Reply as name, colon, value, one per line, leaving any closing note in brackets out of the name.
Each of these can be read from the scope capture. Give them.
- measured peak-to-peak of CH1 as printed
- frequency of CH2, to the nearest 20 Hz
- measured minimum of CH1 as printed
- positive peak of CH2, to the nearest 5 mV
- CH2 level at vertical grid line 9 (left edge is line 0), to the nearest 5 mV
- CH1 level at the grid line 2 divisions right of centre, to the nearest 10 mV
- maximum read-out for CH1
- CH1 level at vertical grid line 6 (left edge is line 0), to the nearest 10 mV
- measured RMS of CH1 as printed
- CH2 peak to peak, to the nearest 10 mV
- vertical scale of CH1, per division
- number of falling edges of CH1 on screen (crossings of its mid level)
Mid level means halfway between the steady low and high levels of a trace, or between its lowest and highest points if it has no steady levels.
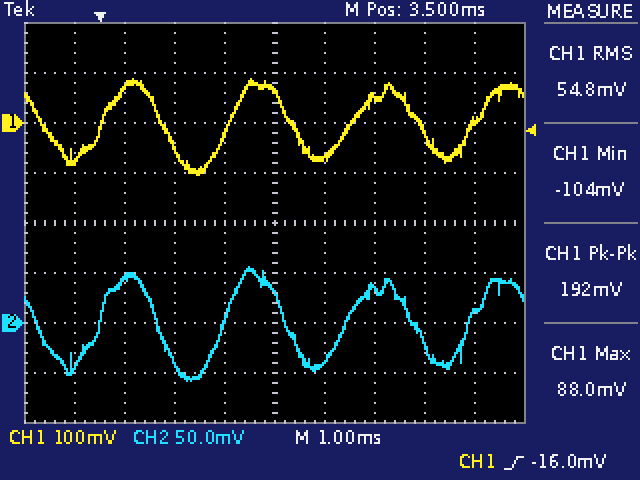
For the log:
measured peak-to-peak of CH1 as printed: 192 mV
frequency of CH2, to the nearest 20 Hz: 400 Hz
measured minimum of CH1 as printed: -104 mV
positive peak of CH2, to the nearest 5 mV: 55 mV
CH2 level at vertical grid line 9 (left edge is line 0), to the nearest 5 mV: 10 mV
CH1 level at the grid line 2 divisions right of centre, to the nearest 10 mV: 50 mV
maximum read-out for CH1: 88.0 mV
CH1 level at vertical grid line 6 (left edge is line 0), to the nearest 10 mV: -70 mV
measured RMS of CH1 as printed: 54.8 mV
CH2 peak to peak, to the nearest 10 mV: 110 mV
vertical scale of CH1, per division: 100 mV
number of falling edges of CH1 on screen: 4
